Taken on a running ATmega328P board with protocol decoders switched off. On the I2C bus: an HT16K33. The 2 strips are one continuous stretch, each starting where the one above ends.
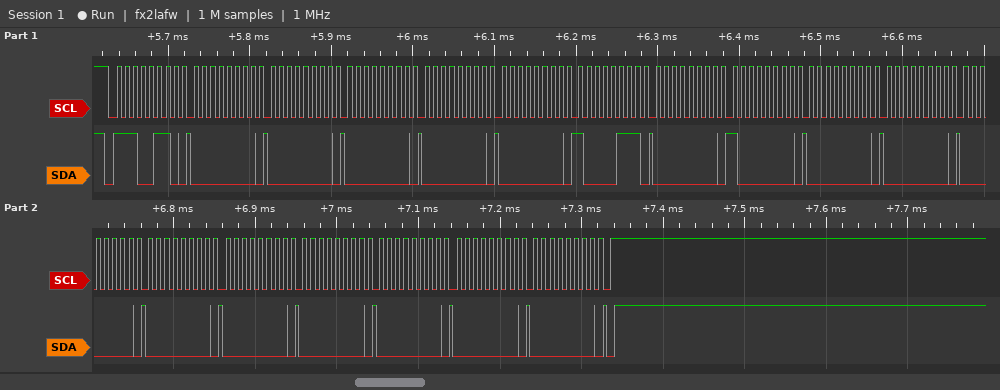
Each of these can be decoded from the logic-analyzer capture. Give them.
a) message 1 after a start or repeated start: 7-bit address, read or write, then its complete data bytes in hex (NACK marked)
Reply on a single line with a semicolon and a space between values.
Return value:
0x73 write: 00 00 00 00 00 87 00 80 00 00 00 00 00 00 00 00 00
